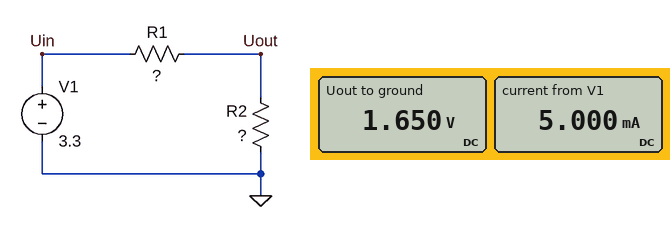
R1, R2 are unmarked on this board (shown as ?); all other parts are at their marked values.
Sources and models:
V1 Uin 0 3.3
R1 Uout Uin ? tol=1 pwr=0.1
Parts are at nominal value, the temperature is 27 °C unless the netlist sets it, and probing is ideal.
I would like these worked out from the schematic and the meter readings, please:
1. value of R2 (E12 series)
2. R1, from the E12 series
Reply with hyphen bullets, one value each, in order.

- 330 Ω
- 330 Ω
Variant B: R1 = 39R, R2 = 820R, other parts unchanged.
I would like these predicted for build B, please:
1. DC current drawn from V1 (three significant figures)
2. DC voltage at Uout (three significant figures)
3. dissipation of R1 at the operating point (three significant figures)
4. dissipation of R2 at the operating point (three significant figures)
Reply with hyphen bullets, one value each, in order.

- 3.84 mA
- 3.15 V
- 576 µW
- 12.1 mW
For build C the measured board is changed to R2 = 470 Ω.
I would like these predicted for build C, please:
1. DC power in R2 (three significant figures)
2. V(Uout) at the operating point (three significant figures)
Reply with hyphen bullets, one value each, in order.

- 8.00 mW
- 1.94 V
